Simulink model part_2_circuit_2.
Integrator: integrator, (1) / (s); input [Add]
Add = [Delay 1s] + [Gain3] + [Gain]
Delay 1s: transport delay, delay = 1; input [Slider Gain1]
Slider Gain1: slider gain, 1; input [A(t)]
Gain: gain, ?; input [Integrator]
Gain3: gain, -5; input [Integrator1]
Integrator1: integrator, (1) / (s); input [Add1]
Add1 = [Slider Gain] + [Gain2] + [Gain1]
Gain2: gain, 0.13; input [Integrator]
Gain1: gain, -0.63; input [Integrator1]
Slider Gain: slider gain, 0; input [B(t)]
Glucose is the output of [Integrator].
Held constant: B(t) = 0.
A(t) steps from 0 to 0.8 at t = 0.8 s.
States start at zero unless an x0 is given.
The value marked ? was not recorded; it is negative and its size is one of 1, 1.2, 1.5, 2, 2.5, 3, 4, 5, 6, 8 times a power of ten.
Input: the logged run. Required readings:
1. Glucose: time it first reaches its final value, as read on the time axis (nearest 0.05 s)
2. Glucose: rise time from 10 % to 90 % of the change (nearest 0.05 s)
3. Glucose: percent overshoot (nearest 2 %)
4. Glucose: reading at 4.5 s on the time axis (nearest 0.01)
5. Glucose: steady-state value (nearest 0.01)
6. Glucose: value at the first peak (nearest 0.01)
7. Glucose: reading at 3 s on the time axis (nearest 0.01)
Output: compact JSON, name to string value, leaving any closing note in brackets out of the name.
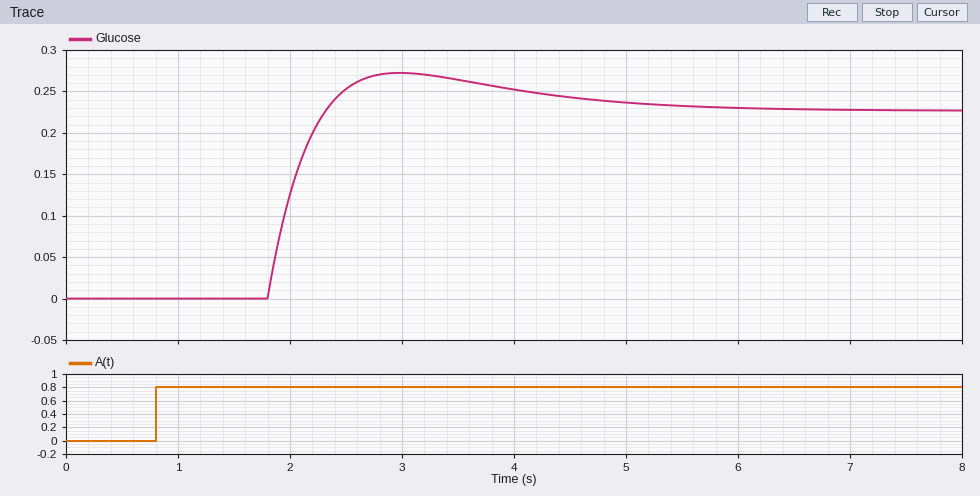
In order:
{"Glucose: time it first reaches its final value, as read on the time axis": "2.30 s", "Glucose: rise time from 10 % to 90 % of the change": "0.40 s", "Glucose: percent overshoot": "20 %", "Glucose: reading at 4.5 s on the time axis": "0.24", "Glucose: steady-state value": "0.23", "Glucose: value at the first peak": "0.27", "Glucose: reading at 3 s on the time axis": "0.27"}
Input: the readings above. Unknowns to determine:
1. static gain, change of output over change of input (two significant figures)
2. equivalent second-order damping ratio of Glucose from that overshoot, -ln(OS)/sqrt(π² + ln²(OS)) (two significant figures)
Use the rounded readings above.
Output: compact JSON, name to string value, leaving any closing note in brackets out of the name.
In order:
{"static gain, change of output over change of input": "0.29", "equivalent second-order damping ratio of Glucose from that overshoot, -ln(OS)/sqrt(π² + ln²(OS))": "0.46"}
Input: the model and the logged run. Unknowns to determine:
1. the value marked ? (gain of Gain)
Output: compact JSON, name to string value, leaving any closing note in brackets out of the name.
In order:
{"the value marked ?": "-2.5"}
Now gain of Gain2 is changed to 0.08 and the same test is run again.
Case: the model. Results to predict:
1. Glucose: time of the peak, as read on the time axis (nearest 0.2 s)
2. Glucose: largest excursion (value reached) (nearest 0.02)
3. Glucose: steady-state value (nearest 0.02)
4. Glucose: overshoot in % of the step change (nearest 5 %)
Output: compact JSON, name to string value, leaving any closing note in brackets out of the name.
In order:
{"Glucose: time of the peak, as read on the time axis": "3.2 s", "Glucose: largest excursion (value reached)": "0.28", "Glucose: steady-state value": "0.26", "Glucose: overshoot in % of the step change": "10 %"}
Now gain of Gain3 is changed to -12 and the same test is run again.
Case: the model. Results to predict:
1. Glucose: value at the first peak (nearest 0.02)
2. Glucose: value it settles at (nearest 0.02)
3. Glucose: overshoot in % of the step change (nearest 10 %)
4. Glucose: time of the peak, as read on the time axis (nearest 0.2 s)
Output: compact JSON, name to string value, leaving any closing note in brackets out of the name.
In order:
{"Glucose: value at the first peak": "0.24", "Glucose: value it settles at": "0.16", "Glucose: overshoot in % of the step change": "50 %", "Glucose: time of the peak, as read on the time axis": "2.6 s"}
